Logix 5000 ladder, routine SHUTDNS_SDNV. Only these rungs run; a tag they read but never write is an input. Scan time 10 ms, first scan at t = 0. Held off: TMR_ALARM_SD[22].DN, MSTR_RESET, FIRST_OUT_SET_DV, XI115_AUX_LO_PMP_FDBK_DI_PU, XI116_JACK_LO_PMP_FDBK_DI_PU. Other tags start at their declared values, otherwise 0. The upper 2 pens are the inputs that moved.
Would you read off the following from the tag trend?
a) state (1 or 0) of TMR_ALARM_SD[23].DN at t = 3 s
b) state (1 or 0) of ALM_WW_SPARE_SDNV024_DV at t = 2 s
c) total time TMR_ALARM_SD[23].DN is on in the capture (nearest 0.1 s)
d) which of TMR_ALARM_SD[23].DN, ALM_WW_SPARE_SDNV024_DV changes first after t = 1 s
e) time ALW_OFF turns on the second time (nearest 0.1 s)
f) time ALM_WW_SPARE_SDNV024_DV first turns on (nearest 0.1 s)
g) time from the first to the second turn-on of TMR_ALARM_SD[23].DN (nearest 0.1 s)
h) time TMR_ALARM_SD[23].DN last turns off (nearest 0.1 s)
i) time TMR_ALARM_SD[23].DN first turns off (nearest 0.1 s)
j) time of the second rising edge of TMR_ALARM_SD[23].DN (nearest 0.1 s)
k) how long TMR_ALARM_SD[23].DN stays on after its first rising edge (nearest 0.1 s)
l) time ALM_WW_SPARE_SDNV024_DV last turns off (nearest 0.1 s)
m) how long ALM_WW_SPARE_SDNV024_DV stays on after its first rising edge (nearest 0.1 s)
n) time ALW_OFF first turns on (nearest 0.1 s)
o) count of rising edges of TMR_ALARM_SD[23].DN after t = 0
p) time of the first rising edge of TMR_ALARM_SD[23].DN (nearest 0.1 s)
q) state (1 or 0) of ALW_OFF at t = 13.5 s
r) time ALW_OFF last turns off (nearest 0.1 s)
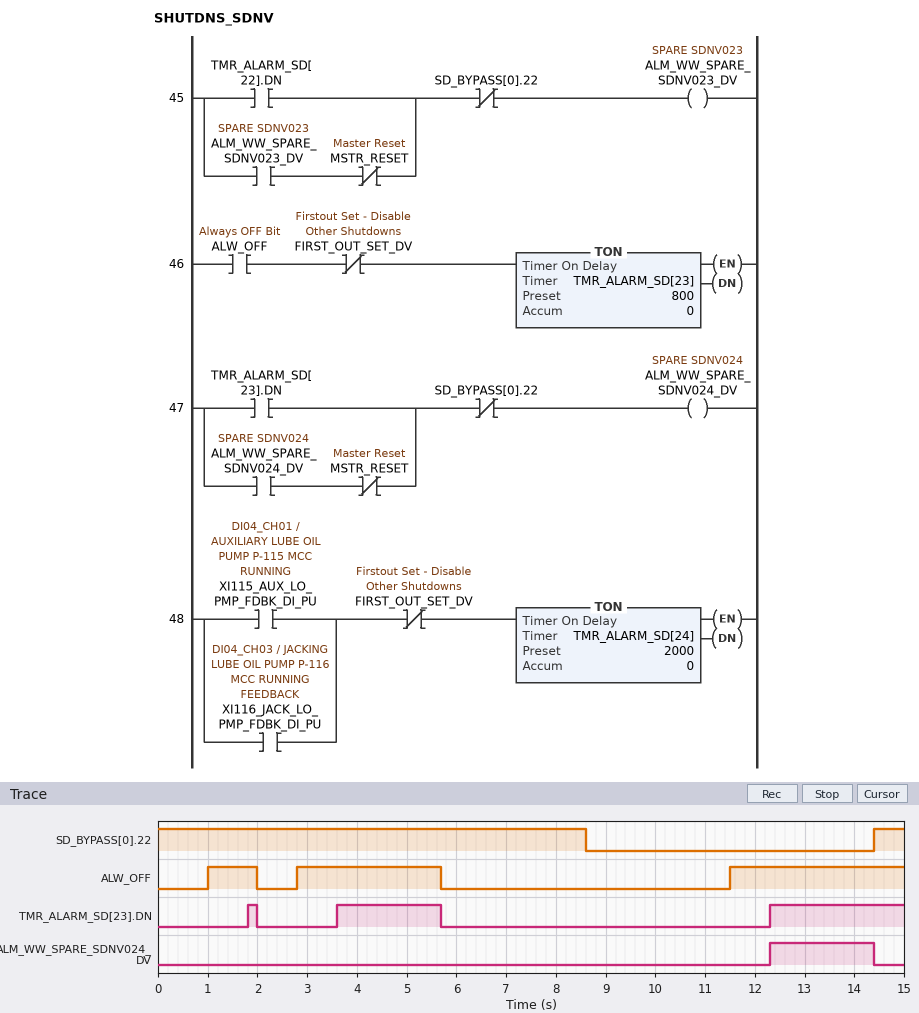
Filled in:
0
0
5.0 s
TMR_ALARM_SD[23].DN
2.8 s
12.3 s
1.8 s
5.7 s
2.0 s
3.6 s
0.2 s
14.4 s
2.1 s
1.0 s
3
1.8 s
1
5.7 s
